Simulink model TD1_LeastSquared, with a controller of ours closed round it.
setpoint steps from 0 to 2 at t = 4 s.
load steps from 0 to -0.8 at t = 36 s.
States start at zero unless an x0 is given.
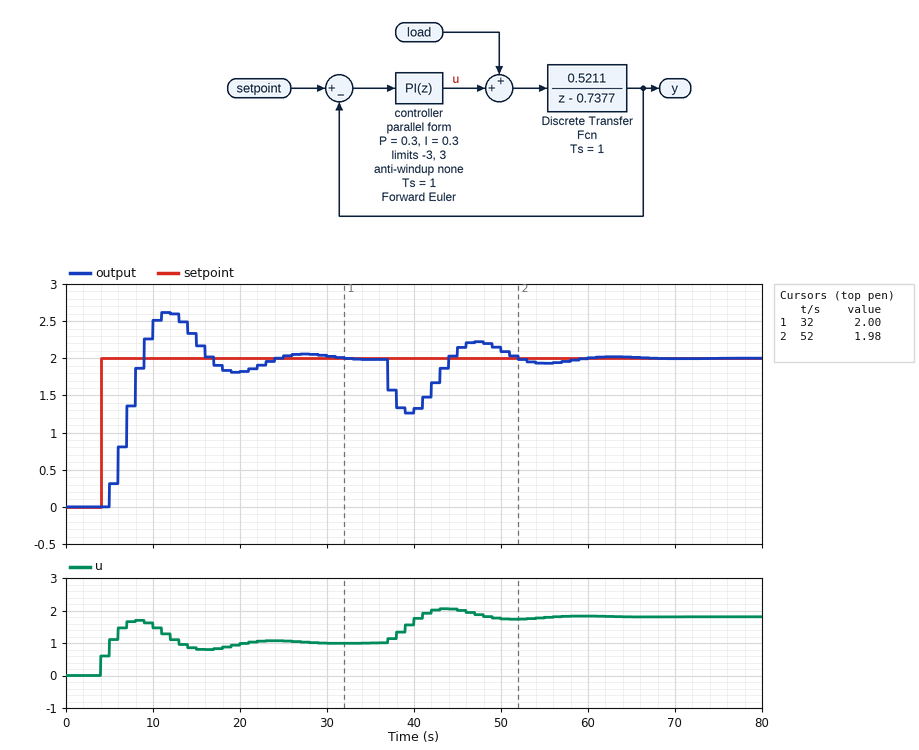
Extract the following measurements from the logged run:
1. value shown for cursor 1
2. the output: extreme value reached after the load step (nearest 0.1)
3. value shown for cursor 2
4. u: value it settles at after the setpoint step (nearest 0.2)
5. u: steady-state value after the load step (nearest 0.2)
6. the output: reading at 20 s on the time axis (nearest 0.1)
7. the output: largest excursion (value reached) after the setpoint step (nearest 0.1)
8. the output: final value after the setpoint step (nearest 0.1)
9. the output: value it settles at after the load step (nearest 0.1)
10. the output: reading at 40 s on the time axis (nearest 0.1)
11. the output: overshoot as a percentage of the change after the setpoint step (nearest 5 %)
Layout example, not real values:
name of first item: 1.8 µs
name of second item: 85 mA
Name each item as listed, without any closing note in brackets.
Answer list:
value shown for cursor 1: 2.00
the output: extreme value reached after the load step: 1.3
value shown for cursor 2: 1.98
u: value it settles at after the setpoint step: 1.0
u: steady-state value after the load step: 1.8
the output: reading at 20 s on the time axis: 1.8
the output: largest excursion (value reached) after the setpoint step: 2.6
the output: final value after the setpoint step: 2.0
the output: value it settles at after the load step: 2.0
the output: reading at 40 s on the time axis: 1.3
the output: overshoot as a percentage of the change after the setpoint step: 30 %
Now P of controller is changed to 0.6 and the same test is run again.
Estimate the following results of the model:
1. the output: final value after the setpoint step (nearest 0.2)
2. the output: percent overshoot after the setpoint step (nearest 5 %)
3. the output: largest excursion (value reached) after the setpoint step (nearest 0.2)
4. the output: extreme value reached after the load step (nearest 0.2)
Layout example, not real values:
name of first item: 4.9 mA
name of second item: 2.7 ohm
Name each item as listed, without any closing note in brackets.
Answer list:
the output: final value after the setpoint step: 2.0
the output: percent overshoot after the setpoint step: 15 %
the output: largest excursion (value reached) after the setpoint step: 2.2
the output: extreme value reached after the load step: 1.4
